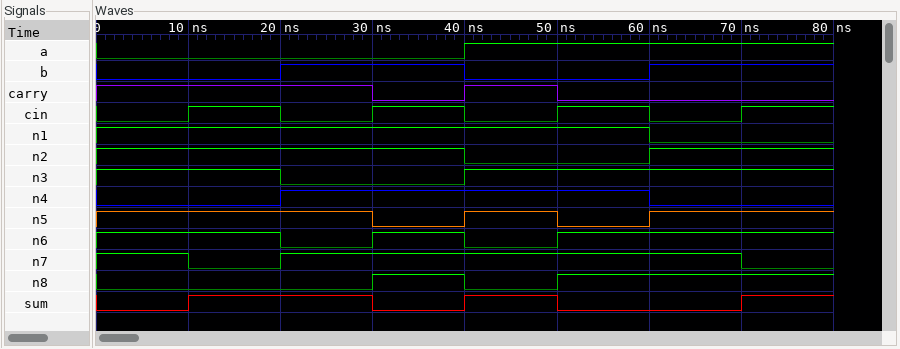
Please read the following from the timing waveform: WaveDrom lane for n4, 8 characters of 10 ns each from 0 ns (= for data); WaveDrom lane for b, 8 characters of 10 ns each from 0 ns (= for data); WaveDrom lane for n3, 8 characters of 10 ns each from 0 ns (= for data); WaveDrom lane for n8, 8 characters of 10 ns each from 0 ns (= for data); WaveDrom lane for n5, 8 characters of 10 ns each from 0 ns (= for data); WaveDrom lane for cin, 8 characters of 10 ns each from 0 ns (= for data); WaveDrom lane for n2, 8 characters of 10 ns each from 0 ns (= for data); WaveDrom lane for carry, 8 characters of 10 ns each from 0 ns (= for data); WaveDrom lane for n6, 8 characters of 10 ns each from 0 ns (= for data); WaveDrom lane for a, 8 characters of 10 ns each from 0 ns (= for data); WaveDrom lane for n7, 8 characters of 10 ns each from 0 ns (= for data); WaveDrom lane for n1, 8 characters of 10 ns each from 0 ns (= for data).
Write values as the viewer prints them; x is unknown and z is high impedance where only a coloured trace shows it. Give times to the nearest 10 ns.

{name: 'n4', wave: '0.1...0.'}
{name: 'b', wave: '0.1.0.1.'}
{name: 'n3', wave: '1.0.1...'}
{name: 'n8', wave: '0..101..'}
{name: 'n5', wave: '1..0101.'}
{name: 'cin', wave: '01010101'}
{name: 'n2', wave: '1...0.1.'}
{name: 'carry', wave: '1..010..'}
{name: 'n6', wave: '1.0101..'}
{name: 'a', wave: '0...1...'}
{name: 'n7', wave: '101....0'}
{name: 'n1', wave: '1.....0.'}
